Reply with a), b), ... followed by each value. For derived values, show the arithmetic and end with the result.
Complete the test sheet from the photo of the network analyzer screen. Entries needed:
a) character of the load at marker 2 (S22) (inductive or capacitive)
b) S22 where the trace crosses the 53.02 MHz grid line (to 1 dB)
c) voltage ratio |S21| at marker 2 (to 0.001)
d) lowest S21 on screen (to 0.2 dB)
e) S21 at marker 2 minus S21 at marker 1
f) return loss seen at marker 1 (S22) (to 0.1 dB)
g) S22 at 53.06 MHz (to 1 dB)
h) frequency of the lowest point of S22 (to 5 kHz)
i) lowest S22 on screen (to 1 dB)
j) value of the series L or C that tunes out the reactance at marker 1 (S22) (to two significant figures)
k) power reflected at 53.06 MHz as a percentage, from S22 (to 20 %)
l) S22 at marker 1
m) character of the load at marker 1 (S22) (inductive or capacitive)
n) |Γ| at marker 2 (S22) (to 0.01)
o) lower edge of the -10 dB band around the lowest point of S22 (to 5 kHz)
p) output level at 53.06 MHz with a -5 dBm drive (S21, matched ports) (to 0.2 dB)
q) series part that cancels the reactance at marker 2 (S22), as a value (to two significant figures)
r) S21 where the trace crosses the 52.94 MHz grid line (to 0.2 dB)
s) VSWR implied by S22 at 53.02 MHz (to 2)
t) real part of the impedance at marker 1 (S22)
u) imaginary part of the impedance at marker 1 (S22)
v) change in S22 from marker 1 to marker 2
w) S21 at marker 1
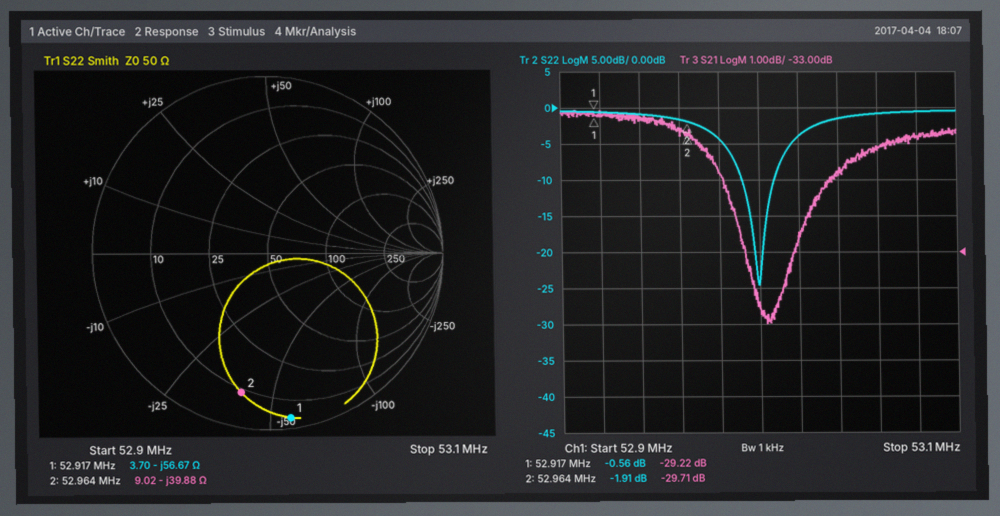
a) capacitive
b) -4 dB
c) 10^(-29.71/20) ≈ 0.033
d) -35.0 dB
e) -29.71 − (-29.22) = -0.49 dB
f) 0.6 dB
g) -1 dB
h) 53.000 MHz
i) -25 dB
j) L = 56.67 Ω/(2π × 52.917 MHz) ≈ 170 nH
k) 10^(-1/10) ≈ 79.4 %, so 80 % to the nearest 20 %
l) -0.56 dB
m) capacitive
n) 0.80
o) 52.990 MHz
p) -5 dBm + (-30.2 dB) = -35.2 dBm
q) L = 39.88 Ω/(2π × 52.964 MHz) ≈ 120 nH
r) -29.2 dB
s) |Γ| = 10^(-4/20) = 0.6310; VSWR = (1 + 0.6310)/(1 − 0.6310) ≈ 4
t) 3.70 Ω
u) -56.67 Ω
v) -1.91 − (-0.56) = -1.35 dB
w) -29.22 dB
